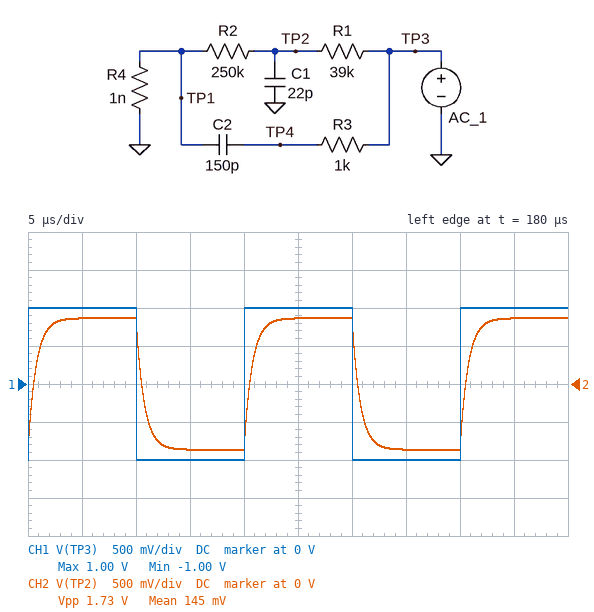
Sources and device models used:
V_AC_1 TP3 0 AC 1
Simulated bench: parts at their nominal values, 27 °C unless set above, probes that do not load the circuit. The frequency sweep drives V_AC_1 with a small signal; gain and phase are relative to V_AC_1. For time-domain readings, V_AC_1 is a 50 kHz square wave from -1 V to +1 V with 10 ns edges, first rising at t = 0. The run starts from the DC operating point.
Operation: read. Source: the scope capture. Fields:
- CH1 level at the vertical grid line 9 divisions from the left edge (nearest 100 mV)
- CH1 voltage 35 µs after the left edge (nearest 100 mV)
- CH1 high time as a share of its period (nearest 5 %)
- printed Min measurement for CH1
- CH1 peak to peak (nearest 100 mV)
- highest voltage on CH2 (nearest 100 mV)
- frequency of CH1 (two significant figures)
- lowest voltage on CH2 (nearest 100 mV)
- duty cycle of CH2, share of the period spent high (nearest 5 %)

1.0 V
-1.0 V
50 %
-1.00 V
2.0 V
900 mV
50 kHz
-900 mV
50 %
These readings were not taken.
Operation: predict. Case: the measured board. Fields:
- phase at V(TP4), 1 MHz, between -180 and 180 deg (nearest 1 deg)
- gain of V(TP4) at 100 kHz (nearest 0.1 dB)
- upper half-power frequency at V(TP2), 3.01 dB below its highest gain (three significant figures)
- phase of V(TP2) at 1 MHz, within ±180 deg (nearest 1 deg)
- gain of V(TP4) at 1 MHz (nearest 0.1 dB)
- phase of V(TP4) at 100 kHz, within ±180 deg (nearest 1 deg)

-43 deg
0 dB
214 kHz
-78 deg
-2.8 dB
-5 deg
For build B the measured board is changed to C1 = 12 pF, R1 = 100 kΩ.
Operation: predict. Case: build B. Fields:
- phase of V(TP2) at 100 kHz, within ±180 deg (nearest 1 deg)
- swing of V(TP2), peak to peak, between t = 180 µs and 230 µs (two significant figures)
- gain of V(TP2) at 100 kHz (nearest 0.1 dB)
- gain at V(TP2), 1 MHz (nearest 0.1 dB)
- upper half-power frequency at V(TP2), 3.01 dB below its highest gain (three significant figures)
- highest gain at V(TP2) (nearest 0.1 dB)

-28 deg
1.4 V
-4.0 dB
-17.7 dB
186 kHz
-2.9 dB
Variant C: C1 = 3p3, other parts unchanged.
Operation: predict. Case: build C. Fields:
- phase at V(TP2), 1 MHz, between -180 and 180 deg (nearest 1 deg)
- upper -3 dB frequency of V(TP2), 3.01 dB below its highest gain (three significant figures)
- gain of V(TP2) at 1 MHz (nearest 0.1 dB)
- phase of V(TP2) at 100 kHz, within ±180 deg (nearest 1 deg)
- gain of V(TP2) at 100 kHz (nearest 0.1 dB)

-35 deg
1.43 MHz
-3.0 dB
-4 deg
-1.3 dB
